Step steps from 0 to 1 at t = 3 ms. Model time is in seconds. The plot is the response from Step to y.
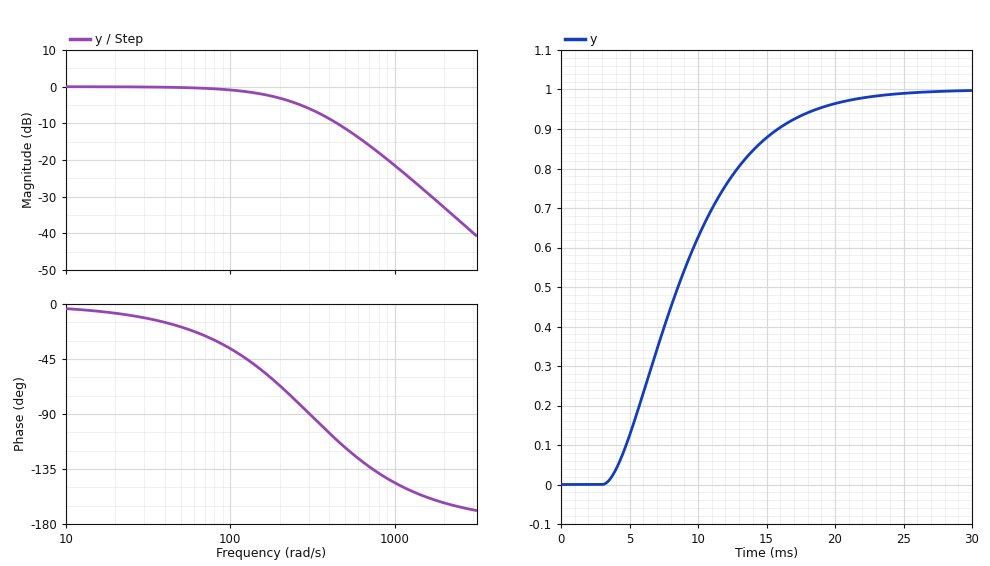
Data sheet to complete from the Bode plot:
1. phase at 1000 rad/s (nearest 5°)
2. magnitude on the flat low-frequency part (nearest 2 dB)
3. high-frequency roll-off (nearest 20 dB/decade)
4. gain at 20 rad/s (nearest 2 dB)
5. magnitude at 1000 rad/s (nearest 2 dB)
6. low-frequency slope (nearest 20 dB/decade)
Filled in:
-145°
0 dB
-40 dB/decade
0 dB
-22 dB
0 dB/decade
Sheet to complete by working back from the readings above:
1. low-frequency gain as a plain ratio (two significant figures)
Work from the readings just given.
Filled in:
1.0
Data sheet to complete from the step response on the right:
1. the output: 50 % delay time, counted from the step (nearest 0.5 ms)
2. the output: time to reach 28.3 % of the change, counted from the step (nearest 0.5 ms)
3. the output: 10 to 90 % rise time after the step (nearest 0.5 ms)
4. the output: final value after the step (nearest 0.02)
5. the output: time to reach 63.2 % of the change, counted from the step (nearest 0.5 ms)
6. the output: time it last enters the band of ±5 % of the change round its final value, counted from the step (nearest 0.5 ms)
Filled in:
5.5 ms
3.5 ms
11.0 ms
1.00
7.0 ms
15.5 ms
